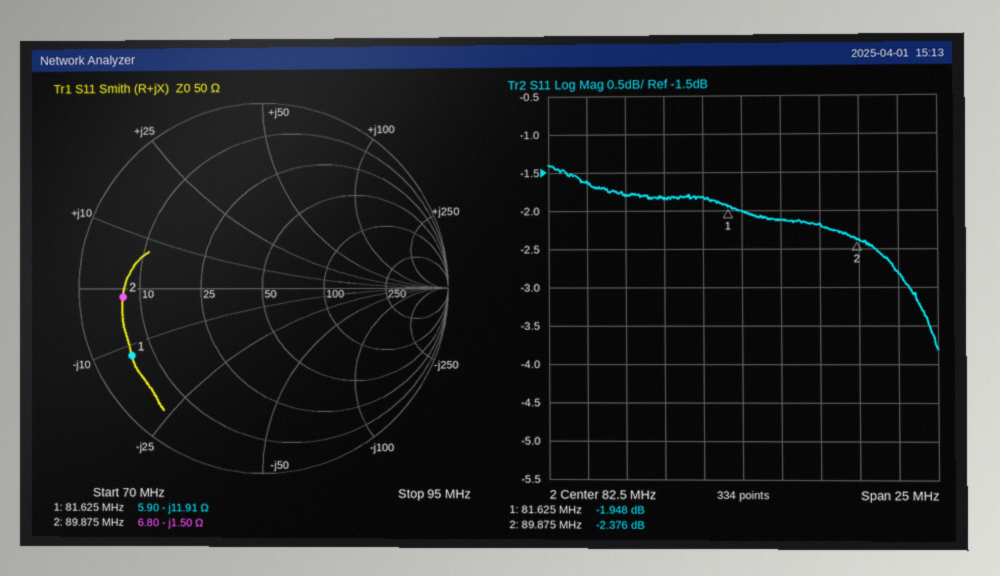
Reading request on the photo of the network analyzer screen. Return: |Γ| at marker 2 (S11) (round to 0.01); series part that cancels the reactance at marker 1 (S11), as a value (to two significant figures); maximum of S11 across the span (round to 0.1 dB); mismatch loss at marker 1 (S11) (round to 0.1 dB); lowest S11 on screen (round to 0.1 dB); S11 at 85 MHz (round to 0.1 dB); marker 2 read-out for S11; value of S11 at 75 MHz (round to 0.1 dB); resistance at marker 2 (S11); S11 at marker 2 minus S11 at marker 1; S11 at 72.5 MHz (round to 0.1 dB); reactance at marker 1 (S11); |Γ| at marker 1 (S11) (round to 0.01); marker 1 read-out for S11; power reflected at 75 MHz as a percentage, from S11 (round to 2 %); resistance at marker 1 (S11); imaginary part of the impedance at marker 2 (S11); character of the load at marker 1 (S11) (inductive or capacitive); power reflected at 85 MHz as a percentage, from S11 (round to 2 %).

0.76
23 nH
-1.4 dB
4.4 dB
-3.8 dB
-2.1 dB
-2.376 dB
-1.8 dB
6.80 Ω
-0.428 dB
-1.6 dB
-11.91 Ω
0.80
-1.948 dB
66 %
5.90 Ω
-1.50 Ω
capacitive
62 %
